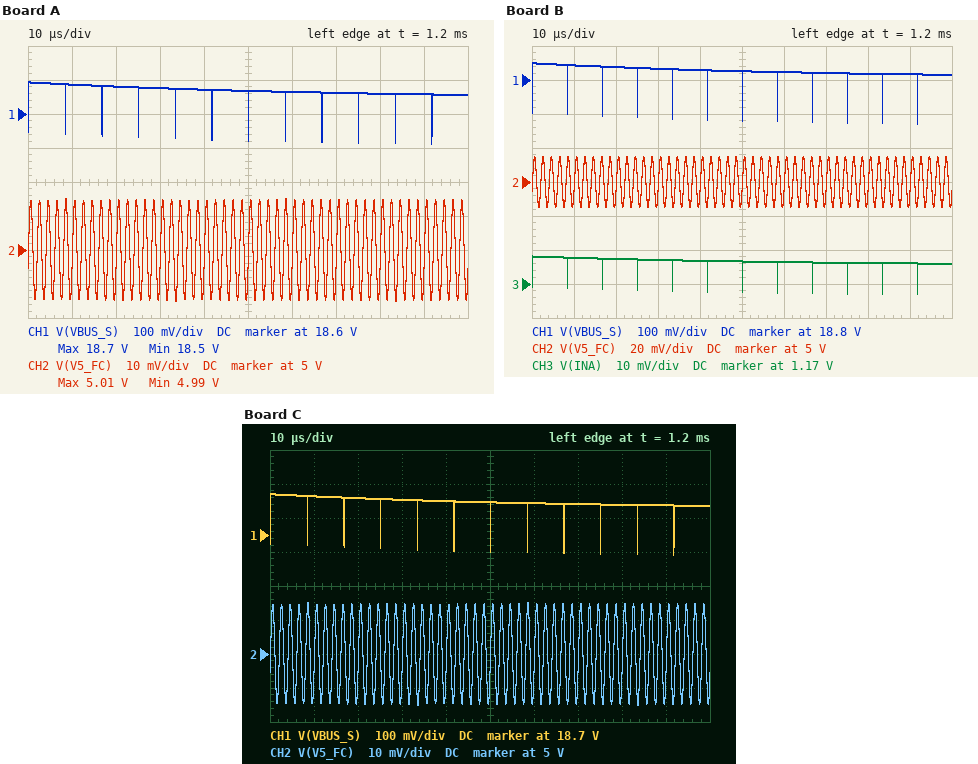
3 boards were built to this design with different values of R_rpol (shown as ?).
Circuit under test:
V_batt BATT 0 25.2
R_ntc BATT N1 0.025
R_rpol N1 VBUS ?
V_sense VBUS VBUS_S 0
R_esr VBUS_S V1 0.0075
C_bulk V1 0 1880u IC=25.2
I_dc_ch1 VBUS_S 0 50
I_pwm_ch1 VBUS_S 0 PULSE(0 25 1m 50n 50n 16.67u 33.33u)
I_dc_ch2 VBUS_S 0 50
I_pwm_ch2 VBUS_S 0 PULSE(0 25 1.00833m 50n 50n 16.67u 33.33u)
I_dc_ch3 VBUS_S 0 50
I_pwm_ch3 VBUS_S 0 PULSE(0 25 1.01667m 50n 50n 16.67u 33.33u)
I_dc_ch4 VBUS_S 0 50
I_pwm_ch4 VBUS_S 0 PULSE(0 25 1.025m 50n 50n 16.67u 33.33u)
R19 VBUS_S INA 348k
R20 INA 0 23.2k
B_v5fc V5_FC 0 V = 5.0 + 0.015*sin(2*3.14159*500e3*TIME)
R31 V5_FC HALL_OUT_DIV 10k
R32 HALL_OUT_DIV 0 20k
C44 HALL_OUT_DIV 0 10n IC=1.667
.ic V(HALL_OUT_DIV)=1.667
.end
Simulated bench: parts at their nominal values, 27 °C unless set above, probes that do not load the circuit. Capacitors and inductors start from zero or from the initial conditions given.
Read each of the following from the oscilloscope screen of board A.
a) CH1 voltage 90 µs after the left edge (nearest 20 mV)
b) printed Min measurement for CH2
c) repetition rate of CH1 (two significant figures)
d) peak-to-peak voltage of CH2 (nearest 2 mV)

18.66 V
4.99 V
120 kHz
30 mV
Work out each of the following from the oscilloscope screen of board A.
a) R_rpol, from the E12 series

1.2 mΩ
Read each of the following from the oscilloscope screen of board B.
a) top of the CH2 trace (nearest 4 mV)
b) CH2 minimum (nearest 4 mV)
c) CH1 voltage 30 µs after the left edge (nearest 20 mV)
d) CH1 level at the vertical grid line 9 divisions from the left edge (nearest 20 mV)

5.016 V
4.984 V
18.84 V
18.82 V
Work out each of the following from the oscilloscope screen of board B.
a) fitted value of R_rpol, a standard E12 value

560 µΩ
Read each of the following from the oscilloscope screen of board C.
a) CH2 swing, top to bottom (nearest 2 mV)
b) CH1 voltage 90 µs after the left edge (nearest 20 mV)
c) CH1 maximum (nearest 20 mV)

30 mV
18.78 V
18.82 V
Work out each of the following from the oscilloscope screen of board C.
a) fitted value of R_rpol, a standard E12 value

680 µΩ
